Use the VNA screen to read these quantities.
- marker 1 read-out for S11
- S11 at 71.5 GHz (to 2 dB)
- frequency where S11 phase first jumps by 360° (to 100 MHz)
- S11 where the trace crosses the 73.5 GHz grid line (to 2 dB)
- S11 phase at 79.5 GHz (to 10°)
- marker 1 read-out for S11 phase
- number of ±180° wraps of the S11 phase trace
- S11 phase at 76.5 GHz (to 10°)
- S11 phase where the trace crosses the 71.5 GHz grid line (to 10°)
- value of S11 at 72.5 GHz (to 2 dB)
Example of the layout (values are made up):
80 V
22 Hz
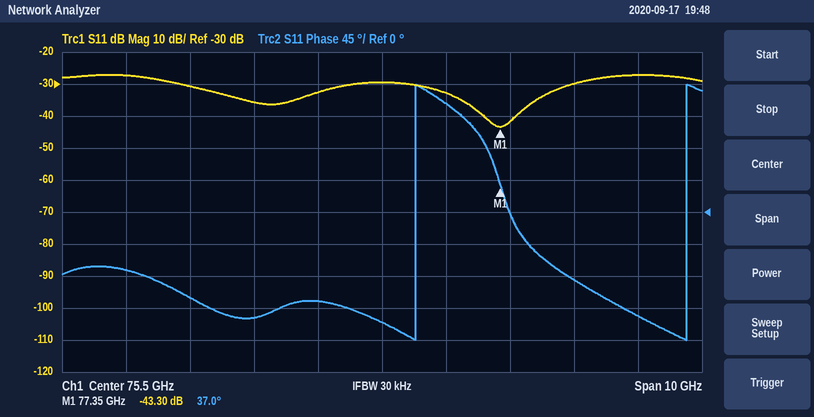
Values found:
-43.30 dB
-28 dB
76.0 GHz
-36 dB
-150°
37.0°
2
150°
-80°
-30 dB
